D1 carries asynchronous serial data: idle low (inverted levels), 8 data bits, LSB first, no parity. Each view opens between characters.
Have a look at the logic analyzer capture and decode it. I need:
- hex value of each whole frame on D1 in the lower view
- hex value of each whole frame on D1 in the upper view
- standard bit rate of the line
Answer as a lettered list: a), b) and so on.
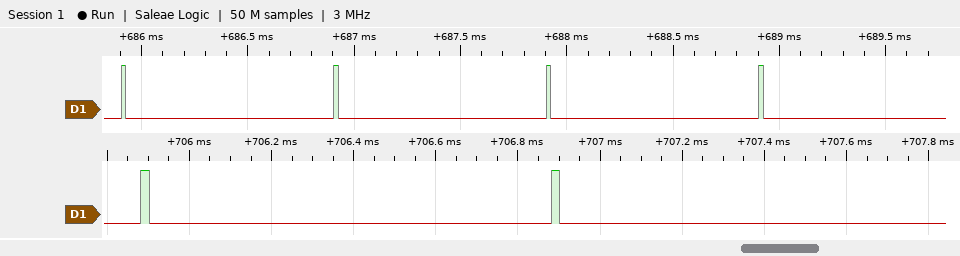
a) FF, FF
b) FF, FF, FF, FF
c) 38400 baud
